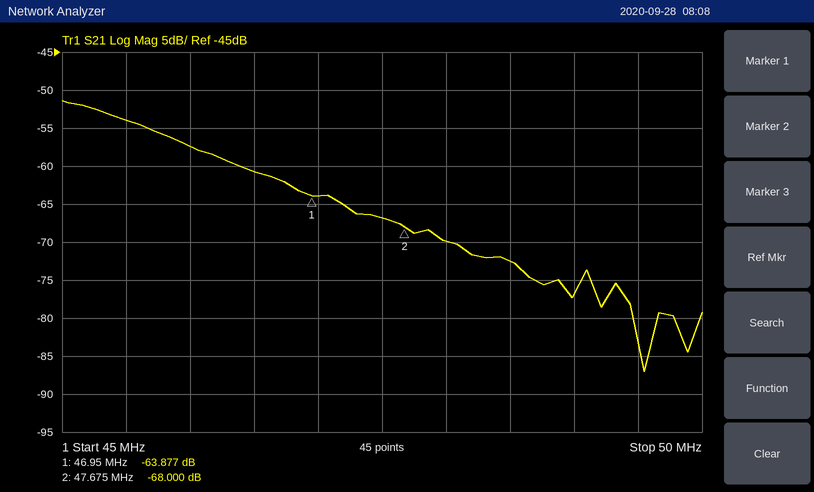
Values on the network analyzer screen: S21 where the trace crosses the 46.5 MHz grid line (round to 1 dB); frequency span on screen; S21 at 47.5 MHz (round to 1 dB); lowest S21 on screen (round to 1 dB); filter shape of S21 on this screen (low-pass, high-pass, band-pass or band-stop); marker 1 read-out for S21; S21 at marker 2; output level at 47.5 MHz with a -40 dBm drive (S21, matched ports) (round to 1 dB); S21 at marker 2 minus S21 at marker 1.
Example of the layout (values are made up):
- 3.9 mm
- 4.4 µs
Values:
- -61 dB
- 5 MHz
- -67 dB
- -87 dB
- low-pass
- -63.877 dB
- -68.000 dB
- -107 dBm
- -4.123 dB
